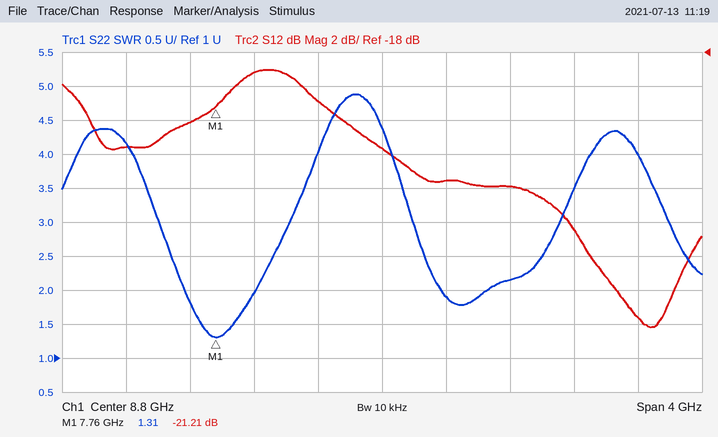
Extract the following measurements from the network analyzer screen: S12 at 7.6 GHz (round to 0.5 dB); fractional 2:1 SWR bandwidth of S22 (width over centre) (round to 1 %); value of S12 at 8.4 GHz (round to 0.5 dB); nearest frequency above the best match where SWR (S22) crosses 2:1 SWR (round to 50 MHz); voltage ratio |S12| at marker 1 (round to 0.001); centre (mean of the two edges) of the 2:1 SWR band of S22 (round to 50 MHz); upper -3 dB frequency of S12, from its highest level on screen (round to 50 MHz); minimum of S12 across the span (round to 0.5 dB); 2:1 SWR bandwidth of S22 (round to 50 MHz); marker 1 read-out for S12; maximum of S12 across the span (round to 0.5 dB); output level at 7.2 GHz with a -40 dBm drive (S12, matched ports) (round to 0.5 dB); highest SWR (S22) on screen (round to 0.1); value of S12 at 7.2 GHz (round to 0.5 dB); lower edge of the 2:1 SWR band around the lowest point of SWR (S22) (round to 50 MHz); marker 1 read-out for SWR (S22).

-22.0 dB
6 %
-21.0 dB
8.00 GHz
0.087
7.80 GHz
8.55 GHz
-34.0 dB
450 MHz
-21.21 dB
-19.0 dB
-63.5 dBm
4.9
-23.5 dB
7.55 GHz
1.31
